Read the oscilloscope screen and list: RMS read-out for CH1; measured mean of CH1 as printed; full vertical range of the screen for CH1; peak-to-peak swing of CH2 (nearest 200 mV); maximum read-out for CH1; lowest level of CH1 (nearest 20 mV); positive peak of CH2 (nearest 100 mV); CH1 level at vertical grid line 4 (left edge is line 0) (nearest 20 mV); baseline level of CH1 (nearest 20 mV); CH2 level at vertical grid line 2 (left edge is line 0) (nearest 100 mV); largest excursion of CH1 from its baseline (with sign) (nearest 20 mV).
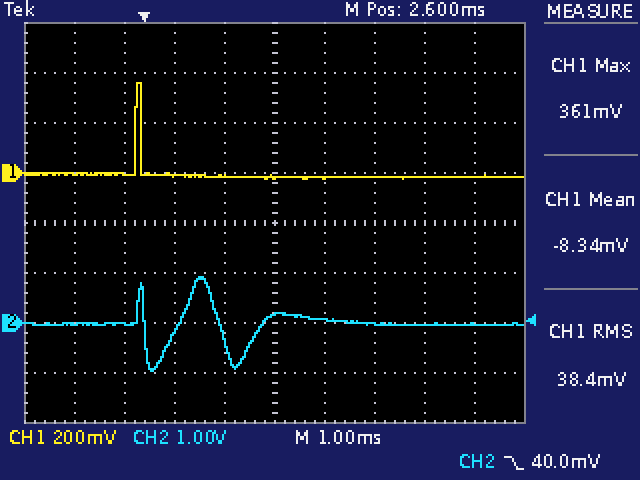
38.4 mV
-8.34 mV
1.6 V
1.8 V
361 mV
-20 mV
900 mV
-20 mV
-20 mV
0.0 V
+380 mV
